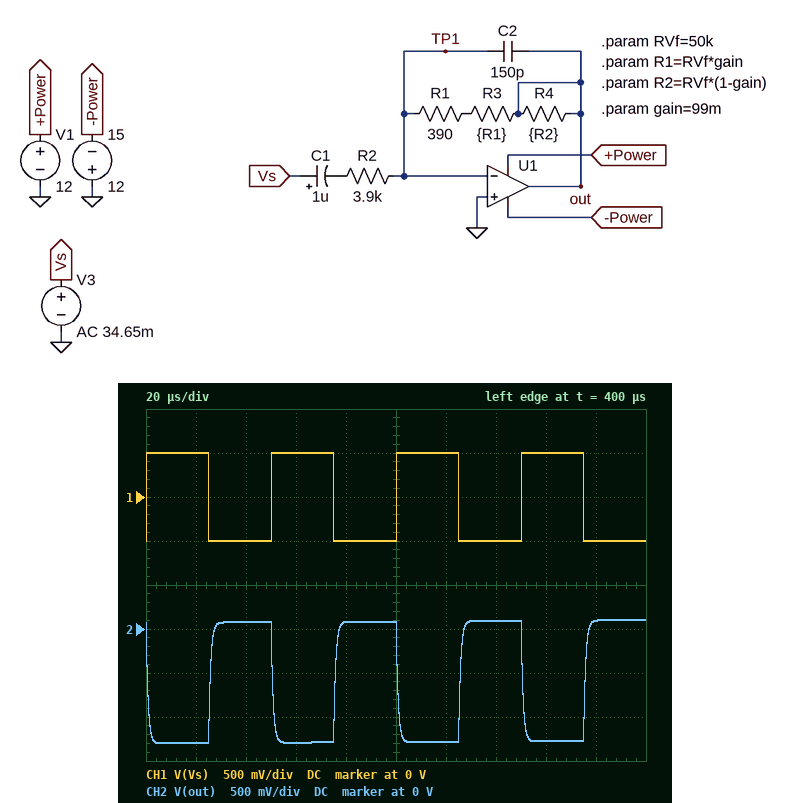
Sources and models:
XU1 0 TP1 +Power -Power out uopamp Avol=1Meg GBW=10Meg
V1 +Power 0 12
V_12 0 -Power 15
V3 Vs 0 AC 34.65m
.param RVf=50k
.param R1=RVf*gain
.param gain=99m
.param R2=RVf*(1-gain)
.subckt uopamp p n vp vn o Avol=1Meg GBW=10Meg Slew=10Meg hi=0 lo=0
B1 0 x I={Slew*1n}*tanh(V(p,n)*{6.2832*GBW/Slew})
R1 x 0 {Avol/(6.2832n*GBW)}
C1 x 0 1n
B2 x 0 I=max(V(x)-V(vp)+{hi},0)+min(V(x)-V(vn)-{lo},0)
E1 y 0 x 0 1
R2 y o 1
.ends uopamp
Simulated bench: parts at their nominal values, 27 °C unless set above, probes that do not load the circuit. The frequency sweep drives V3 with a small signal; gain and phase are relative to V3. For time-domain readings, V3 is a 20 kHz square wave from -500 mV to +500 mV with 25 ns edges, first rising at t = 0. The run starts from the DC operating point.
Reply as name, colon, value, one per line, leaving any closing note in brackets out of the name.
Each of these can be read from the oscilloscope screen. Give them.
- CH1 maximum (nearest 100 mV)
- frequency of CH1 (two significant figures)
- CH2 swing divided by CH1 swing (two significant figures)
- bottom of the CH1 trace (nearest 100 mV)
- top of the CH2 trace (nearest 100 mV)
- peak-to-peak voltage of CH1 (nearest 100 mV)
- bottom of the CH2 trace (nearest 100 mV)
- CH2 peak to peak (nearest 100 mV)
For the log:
CH1 maximum: 500 mV
frequency of CH1: 20 kHz
CH2 swing divided by CH1 swing: 1.4
bottom of the CH1 trace: -500 mV
top of the CH2 trace: 100 mV
peak-to-peak voltage of CH1: 1.0 V
bottom of the CH2 trace: -1.3 V
CH2 peak to peak: 1.4 V
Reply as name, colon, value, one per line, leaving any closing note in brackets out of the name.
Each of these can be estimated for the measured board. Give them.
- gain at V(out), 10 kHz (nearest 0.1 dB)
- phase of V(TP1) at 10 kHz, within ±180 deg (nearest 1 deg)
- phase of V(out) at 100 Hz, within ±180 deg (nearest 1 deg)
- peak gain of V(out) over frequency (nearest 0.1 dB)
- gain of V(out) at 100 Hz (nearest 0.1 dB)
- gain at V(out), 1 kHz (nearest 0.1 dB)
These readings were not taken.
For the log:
gain at V(out), 10 kHz: 2.7 dB
phase of V(TP1) at 10 kHz, within ±180 deg: 87 deg
phase of V(out) at 100 Hz, within ±180 deg: -158 deg
peak gain of V(out) over frequency: 2.7 dB
gain of V(out) at 100 Hz: 2.1 dB
gain at V(out), 1 kHz: 2.7 dB
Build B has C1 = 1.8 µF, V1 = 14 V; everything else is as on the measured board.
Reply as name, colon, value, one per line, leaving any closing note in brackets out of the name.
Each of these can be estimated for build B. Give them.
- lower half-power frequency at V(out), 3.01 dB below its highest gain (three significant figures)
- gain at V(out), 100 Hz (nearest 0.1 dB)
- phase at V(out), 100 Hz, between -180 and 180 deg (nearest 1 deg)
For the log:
lower half-power frequency at V(out), 3.01 dB below its highest gain: 22.7 Hz
gain at V(out), 100 Hz: 2.5 dB
phase at V(out), 100 Hz, between -180 and 180 deg: -167 deg
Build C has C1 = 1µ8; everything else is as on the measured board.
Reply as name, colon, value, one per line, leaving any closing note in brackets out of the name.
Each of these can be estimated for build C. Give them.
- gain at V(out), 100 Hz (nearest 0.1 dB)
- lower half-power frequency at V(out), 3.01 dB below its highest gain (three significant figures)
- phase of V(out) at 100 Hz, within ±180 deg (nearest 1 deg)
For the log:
gain at V(out), 100 Hz: 2.5 dB
lower half-power frequency at V(out), 3.01 dB below its highest gain: 22.7 Hz
phase of V(out) at 100 Hz, within ±180 deg: -167 deg
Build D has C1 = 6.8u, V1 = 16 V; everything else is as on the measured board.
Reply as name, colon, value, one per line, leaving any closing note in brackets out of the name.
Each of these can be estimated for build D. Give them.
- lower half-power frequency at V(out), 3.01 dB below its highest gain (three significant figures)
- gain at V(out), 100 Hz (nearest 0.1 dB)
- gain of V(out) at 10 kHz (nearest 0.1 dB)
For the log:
lower half-power frequency at V(out), 3.01 dB below its highest gain: 6.00 Hz
gain at V(out), 100 Hz: 2.7 dB
gain of V(out) at 10 kHz: 2.7 dB
